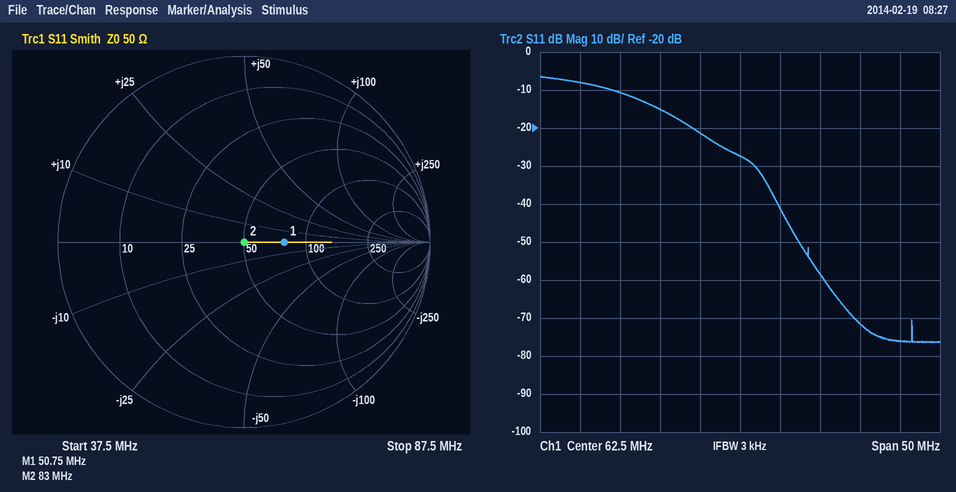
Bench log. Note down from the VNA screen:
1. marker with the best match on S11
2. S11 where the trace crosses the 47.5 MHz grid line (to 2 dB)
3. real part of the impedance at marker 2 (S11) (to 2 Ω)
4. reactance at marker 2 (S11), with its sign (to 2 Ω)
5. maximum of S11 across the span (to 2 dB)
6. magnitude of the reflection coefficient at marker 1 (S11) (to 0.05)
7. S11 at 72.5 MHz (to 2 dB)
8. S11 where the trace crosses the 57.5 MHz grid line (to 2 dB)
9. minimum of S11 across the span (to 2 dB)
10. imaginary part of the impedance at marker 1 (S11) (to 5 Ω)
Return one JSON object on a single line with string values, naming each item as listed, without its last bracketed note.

{"marker with the best match on S11": "marker 2", "S11 where the trace crosses the 47.5 MHz grid line": "-10 dB", "real part of the impedance at marker 2 (S11)": "50 Ω", "reactance at marker 2 (S11), with its sign": "0 Ω", "maximum of S11 across the span": "-6 dB", "magnitude of the reflection coefficient at marker 1 (S11)": "0.20", "S11 at 72.5 MHz": "-58 dB", "S11 where the trace crosses the 57.5 MHz grid line": "-22 dB", "minimum of S11 across the span": "-76 dB", "imaginary part of the impedance at marker 1 (S11)": "0 Ω"}
